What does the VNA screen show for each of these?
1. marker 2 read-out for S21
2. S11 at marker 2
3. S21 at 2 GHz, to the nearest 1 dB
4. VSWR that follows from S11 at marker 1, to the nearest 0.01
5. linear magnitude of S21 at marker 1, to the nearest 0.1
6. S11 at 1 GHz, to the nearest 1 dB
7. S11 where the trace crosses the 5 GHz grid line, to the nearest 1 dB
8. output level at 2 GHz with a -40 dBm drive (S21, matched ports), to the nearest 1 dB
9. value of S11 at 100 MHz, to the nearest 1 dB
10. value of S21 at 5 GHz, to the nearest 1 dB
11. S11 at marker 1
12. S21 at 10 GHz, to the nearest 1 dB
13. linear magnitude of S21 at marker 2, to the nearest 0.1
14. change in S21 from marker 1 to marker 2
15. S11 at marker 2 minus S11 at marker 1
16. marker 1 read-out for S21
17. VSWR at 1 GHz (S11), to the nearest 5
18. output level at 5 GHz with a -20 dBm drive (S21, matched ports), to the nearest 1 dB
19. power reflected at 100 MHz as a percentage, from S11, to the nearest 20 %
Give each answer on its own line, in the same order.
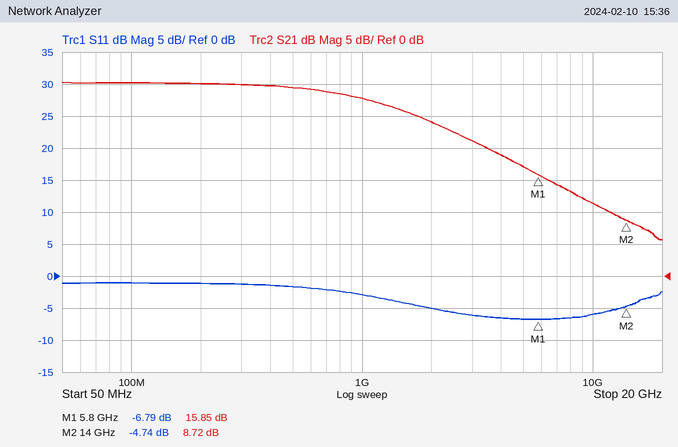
8.72 dB
-4.74 dB
24 dB
2.69
6.2
-3 dB
-7 dB
-16 dBm
-1 dB
17 dB
-6.79 dB
11 dB
2.7
-7.13 dB
2.05 dB
15.85 dB
5
-3 dBm
80 %
